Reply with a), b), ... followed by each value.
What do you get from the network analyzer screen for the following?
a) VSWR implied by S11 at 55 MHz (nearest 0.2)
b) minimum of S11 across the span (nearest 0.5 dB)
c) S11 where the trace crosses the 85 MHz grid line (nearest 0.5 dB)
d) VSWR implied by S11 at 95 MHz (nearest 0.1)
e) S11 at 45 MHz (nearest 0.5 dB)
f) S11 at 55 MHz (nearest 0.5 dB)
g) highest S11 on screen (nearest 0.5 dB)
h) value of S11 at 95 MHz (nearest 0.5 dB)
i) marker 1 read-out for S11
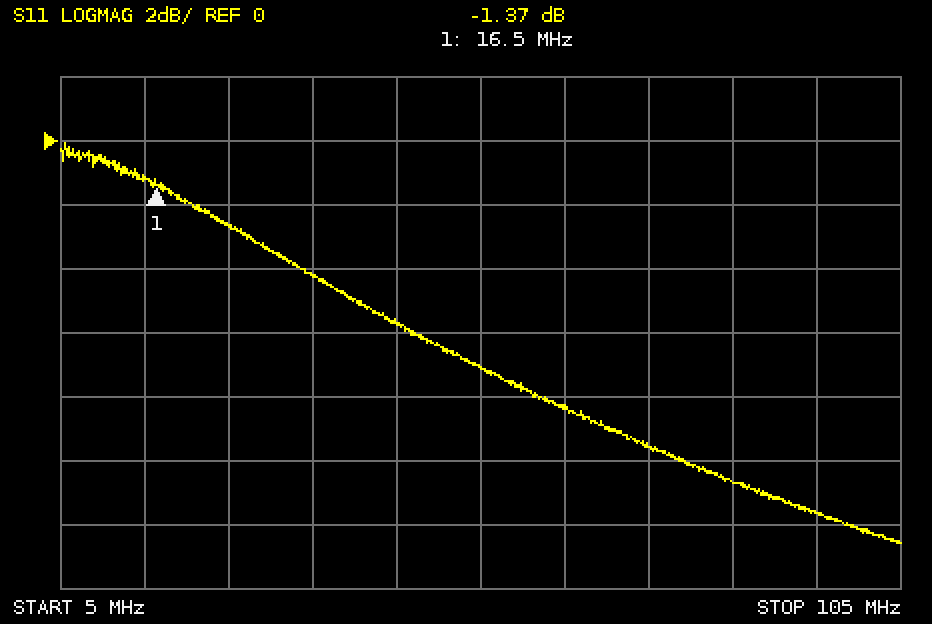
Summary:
a) 2.6
b) -12.5 dB
c) -10.5 dB
d) 1.7
e) -5.5 dB
f) -7.0 dB
g) 0.0 dB
h) -11.5 dB
i) -1.37 dB
